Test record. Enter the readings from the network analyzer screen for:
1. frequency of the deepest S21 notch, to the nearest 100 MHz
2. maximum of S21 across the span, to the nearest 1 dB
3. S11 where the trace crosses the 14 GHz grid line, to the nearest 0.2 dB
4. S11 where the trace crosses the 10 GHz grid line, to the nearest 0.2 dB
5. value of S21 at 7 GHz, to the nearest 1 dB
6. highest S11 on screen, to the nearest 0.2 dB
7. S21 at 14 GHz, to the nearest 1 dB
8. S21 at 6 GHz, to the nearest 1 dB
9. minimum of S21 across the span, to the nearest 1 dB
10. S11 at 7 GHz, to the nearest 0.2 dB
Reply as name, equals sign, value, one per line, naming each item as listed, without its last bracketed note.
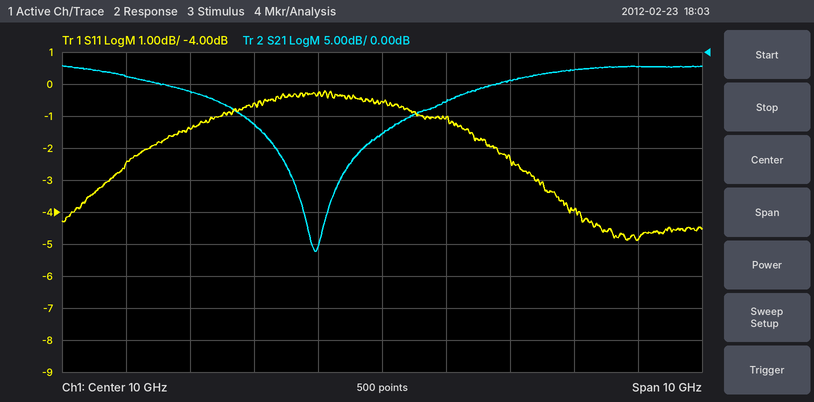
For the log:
frequency of the deepest S21 notch, to the nearest 100 MHz = 9.0 GHz
maximum of S21 across the span, to the nearest 1 dB = -2 dB
S11 where the trace crosses the 14 GHz grid line, to the nearest 0.2 dB = -4.8 dB
S11 where the trace crosses the 10 GHz grid line, to the nearest 0.2 dB = -0.6 dB
value of S21 at 7 GHz, to the nearest 1 dB = -6 dB
highest S11 on screen, to the nearest 0.2 dB = -0.2 dB
S21 at 14 GHz, to the nearest 1 dB = -2 dB
S21 at 6 GHz, to the nearest 1 dB = -4 dB
minimum of S21 across the span, to the nearest 1 dB = -31 dB
S11 at 7 GHz, to the nearest 0.2 dB = -1.4 dB
